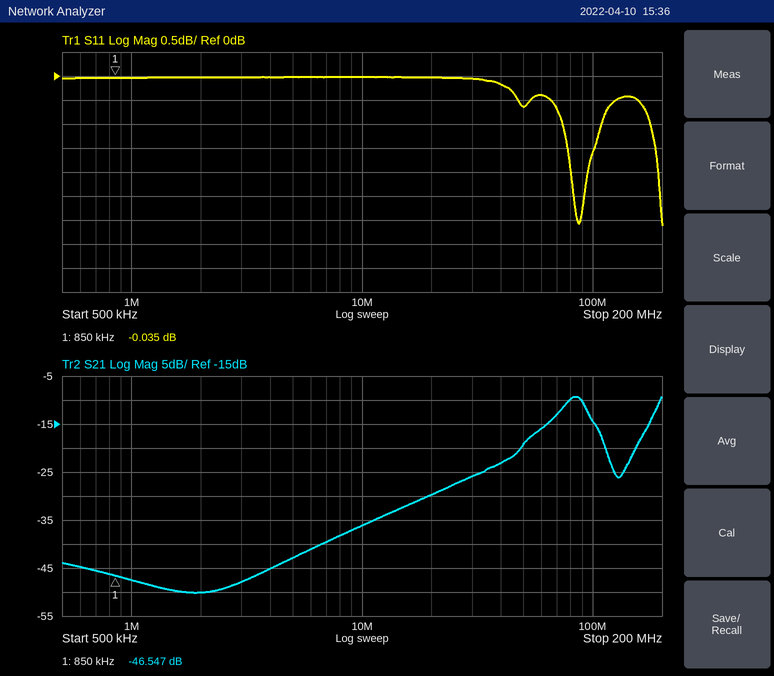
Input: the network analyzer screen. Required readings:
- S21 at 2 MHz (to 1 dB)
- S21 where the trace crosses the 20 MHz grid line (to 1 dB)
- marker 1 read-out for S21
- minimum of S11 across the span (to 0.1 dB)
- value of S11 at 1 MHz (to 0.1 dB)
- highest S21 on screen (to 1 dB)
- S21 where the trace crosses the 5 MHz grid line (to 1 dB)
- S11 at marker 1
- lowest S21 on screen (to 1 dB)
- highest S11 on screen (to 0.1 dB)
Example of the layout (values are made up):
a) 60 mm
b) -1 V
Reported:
a) -50 dB
b) -30 dB
c) -46.547 dB
d) -3.1 dB
e) 0.0 dB
f) -9 dB
g) -43 dB
h) -0.035 dB
i) -50 dB
j) 0.0 dB
